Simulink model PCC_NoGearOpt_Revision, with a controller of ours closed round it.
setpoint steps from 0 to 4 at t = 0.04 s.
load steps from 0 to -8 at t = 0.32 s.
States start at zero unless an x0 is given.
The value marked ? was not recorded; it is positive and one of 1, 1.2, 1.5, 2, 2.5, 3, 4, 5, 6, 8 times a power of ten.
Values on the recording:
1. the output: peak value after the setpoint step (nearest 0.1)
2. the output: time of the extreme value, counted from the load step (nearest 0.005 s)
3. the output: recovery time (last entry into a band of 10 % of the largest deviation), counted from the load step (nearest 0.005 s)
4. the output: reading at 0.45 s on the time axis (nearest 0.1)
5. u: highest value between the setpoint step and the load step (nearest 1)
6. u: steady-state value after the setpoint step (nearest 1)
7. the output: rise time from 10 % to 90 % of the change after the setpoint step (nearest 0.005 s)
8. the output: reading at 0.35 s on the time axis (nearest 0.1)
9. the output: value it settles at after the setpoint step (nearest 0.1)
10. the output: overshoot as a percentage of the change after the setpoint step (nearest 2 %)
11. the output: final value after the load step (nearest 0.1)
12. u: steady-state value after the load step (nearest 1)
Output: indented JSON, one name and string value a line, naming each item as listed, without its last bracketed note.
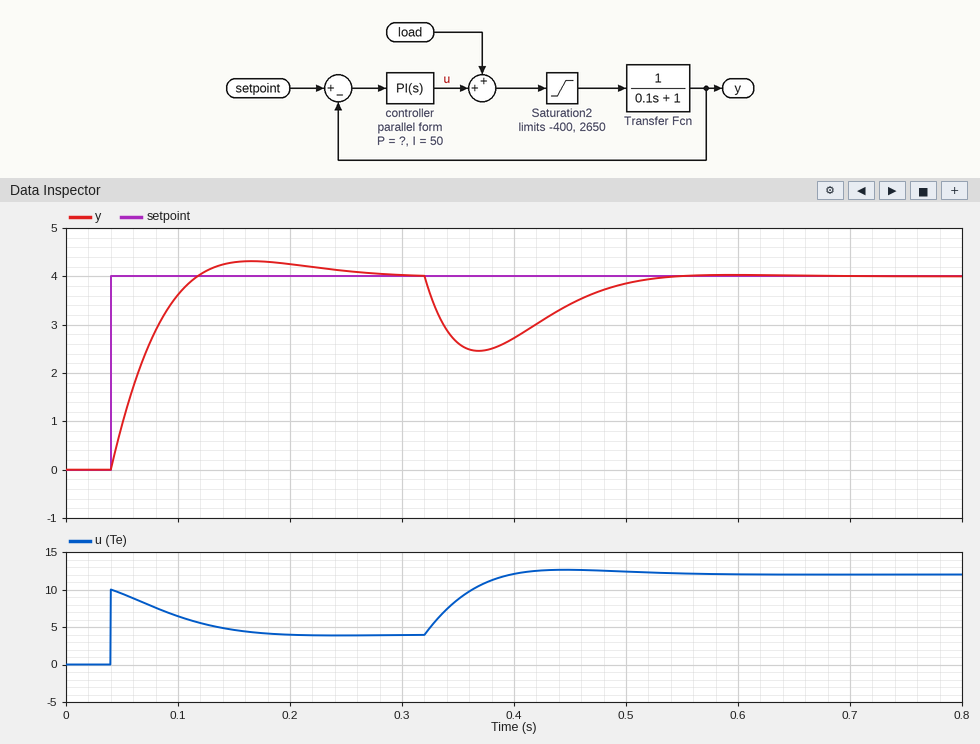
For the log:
{
  "the output: peak value after the setpoint step": "4.3",
  "the output: time of the extreme value, counted from the load step": "0.050 s",
  "the output: recovery time (last entry into a band of 10 % of the largest deviation), counted from the load step": "0.180 s",
  "the output: reading at 0.45 s on the time axis": "3.4",
  "u: highest value between the setpoint step and the load step": "10",
  "u: steady-state value after the setpoint step": "4",
  "the output: rise time from 10 % to 90 % of the change after the setpoint step": "0.055 s",
  "the output: reading at 0.35 s on the time axis": "2.6",
  "the output: value it settles at after the setpoint step": "4.0",
  "the output: overshoot as a percentage of the change after the setpoint step": "8 %",
  "the output: final value after the load step": "4.0",
  "u: steady-state value after the load step": "12"
}
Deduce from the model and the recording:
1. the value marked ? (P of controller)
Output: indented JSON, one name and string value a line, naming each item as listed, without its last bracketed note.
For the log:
{
  "the value marked ?": "2.5"
}
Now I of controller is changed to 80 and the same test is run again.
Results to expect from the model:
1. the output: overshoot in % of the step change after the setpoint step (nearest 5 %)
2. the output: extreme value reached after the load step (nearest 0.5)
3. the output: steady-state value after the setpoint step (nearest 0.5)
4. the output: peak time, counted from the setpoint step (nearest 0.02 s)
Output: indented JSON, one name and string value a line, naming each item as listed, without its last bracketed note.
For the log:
{
  "the output: overshoot in % of the step change after the setpoint step": "15 %",
  "the output: extreme value reached after the load step": "2.5",
  "the output: steady-state value after the setpoint step": "4.0",
  "the output: peak time, counted from the setpoint step": "0.10 s"
}
